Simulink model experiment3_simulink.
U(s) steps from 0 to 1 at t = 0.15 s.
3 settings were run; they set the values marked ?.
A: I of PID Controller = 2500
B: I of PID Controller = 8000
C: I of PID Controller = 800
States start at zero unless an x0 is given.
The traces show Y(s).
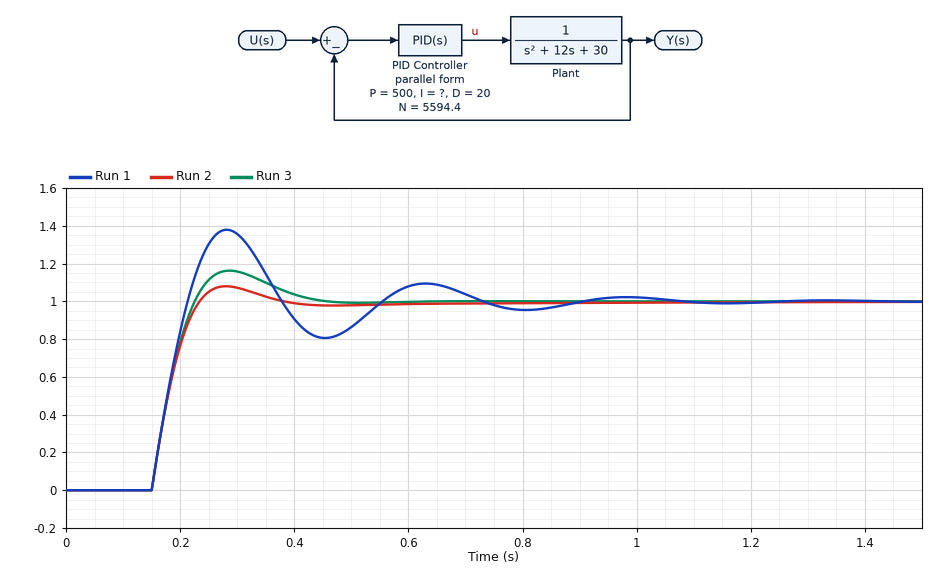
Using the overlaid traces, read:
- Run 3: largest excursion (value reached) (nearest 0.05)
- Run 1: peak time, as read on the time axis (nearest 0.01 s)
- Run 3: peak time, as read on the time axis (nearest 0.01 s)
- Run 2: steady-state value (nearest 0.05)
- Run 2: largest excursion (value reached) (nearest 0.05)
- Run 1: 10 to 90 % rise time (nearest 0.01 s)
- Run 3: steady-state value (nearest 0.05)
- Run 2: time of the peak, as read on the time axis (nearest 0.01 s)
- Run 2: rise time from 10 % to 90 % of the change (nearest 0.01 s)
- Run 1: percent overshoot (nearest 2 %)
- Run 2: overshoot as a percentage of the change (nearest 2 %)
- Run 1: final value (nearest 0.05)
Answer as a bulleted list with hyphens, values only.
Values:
- 1.15
- 0.28 s
- 0.29 s
- 1.00
- 1.10
- 0.05 s
- 1.00
- 0.28 s
- 0.06 s
- 38 %
- 8 %
- 1.00
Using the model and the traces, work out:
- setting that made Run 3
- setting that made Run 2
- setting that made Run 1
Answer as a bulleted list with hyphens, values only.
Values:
- A
- C
- B
